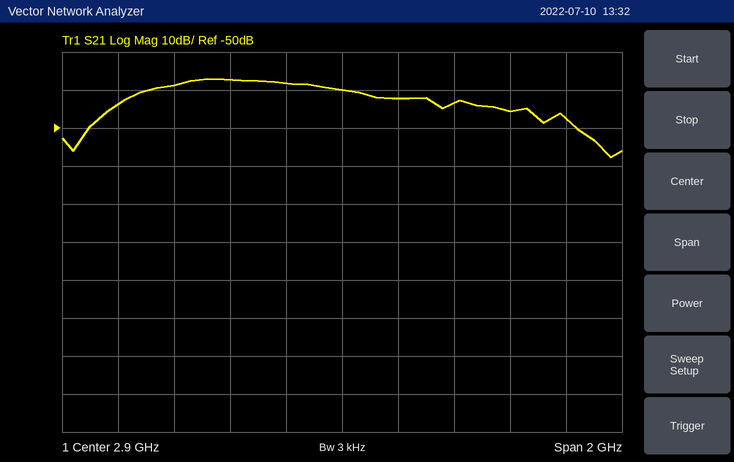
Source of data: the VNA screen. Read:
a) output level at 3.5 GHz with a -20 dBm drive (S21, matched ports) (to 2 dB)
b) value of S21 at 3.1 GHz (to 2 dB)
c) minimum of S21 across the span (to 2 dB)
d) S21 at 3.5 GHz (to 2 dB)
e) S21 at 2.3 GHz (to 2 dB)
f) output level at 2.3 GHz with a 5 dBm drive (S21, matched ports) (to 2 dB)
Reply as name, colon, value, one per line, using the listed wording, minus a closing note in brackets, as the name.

output level at 3.5 GHz with a -20 dBm drive (S21, matched ports): -66 dBm
value of S21 at 3.1 GHz: -42 dB
minimum of S21 across the span: -58 dB
S21 at 3.5 GHz: -46 dB
S21 at 2.3 GHz: -38 dB
output level at 2.3 GHz with a 5 dBm drive (S21, matched ports): -34 dBm
